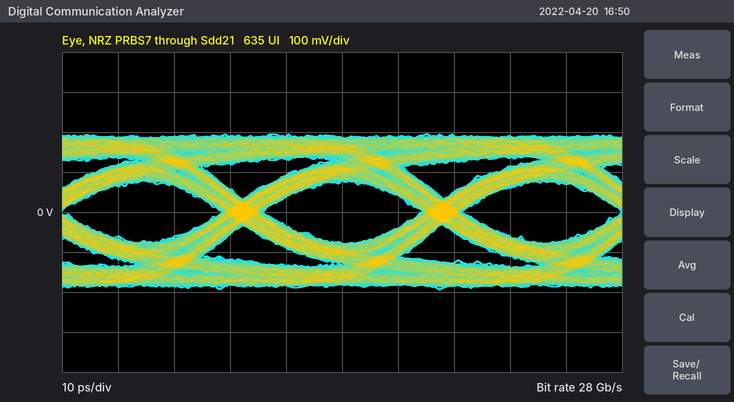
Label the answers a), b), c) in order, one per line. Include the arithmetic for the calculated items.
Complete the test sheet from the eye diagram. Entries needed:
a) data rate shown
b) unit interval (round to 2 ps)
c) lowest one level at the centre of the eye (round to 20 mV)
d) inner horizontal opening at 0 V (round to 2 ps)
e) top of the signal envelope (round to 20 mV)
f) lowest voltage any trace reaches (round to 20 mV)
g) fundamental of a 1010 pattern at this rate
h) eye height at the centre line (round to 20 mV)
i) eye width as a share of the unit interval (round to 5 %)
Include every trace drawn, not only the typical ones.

a) 28 Gb/s
b) 36 ps
c) 80 mV
d) 28 ps
e) 200 mV
f) -200 mV
g) 14 GHz
h) 160 mV
i) 28 ps / 36 ps ≈ 77.8 %, so 80 % to the nearest 5 %
